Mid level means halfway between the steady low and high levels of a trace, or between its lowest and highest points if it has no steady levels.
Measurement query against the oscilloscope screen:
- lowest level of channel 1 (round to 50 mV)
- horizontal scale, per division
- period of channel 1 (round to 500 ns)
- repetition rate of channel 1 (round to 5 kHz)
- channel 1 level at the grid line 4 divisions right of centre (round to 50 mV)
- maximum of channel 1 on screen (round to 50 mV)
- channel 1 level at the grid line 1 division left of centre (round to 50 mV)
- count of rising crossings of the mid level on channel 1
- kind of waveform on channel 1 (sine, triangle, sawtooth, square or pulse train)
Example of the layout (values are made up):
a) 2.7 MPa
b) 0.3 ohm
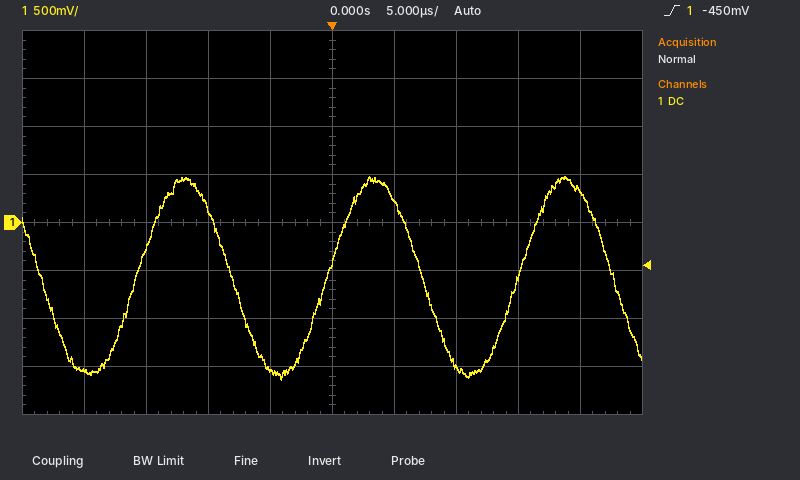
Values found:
a) -1.65 V
b) 5 µs
c) 15.5 µs
d) 65 kHz
e) 350 mV
f) 500 mV
g) -1.55 V
h) 3
i) sine
